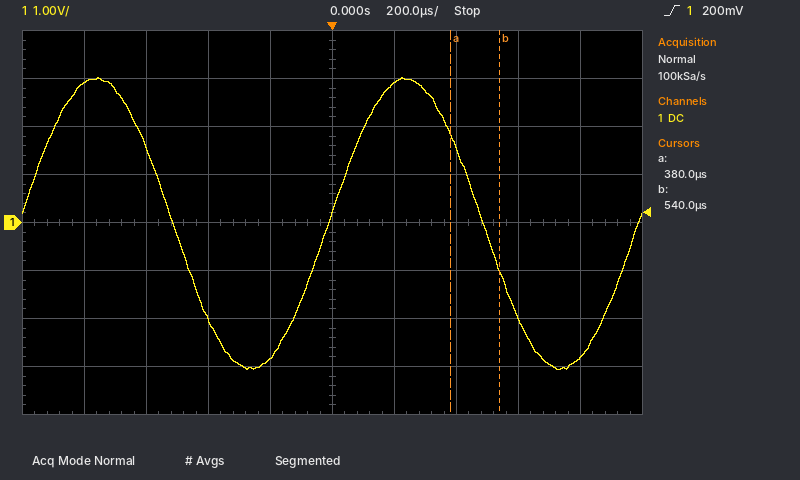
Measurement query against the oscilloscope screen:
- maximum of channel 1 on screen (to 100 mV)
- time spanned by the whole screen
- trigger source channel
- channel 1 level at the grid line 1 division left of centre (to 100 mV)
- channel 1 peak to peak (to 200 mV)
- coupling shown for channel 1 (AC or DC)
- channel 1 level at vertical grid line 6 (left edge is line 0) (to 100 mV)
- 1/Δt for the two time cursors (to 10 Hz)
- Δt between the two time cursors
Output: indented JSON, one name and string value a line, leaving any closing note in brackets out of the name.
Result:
{
  "maximum of channel 1 on screen": "3.0 V",
  "time spanned by the whole screen": "2 ms",
  "trigger source channel": "channel 1",
  "channel 1 level at the grid line 1 division left of centre": "-2.8 V",
  "channel 1 peak to peak": "6.0 V",
  "coupling shown for channel 1": "DC",
  "channel 1 level at vertical grid line 6 (left edge is line 0)": "2.9 V",
  "1/Δt for the two time cursors": "6.25 kHz",
  "Δt between the two time cursors": "160 µs"
}
